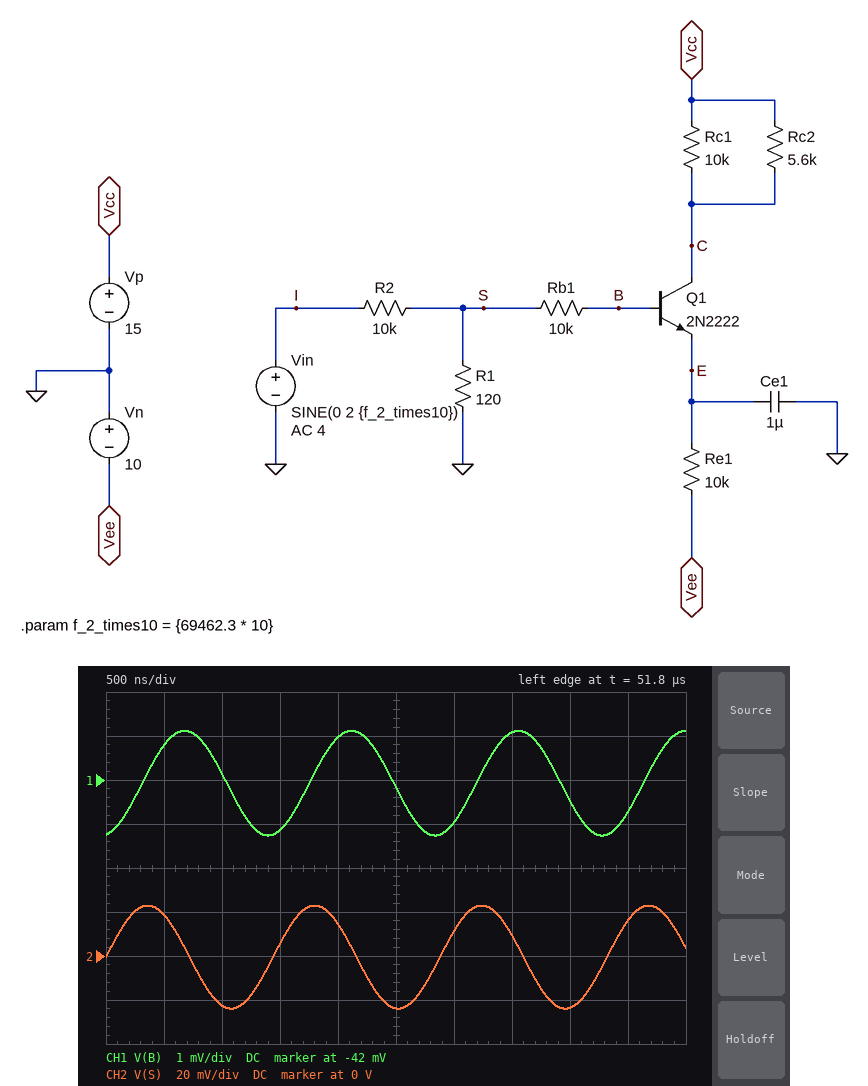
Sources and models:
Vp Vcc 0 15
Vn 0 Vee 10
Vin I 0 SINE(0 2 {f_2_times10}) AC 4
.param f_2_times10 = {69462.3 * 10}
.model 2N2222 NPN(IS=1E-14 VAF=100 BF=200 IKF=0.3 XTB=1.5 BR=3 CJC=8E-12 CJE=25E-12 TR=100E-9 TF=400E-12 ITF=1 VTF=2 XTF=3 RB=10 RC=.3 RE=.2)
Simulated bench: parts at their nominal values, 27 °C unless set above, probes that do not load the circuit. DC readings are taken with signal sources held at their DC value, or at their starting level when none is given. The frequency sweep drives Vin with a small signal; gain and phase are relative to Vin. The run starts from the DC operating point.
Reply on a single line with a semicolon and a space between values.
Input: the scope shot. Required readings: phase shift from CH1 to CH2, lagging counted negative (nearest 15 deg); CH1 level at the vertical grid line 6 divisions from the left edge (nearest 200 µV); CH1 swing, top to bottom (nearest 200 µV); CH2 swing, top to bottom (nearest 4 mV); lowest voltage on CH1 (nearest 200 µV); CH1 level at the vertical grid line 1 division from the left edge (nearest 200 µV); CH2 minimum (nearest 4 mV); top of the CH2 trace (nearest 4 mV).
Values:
75 deg; -43.0 mV; 2.4 mV; 48 mV; -43.2 mV; -41.2 mV; -24 mV; 24 mV
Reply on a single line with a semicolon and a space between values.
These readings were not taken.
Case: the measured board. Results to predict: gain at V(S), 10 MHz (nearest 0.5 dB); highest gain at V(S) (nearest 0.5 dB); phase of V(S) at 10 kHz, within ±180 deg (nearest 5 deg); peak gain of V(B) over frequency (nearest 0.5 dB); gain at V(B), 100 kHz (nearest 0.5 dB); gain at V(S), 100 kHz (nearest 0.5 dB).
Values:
-38.5 dB; -38.5 dB; 0 deg; -38.5 dB; -50.0 dB; -38.5 dB
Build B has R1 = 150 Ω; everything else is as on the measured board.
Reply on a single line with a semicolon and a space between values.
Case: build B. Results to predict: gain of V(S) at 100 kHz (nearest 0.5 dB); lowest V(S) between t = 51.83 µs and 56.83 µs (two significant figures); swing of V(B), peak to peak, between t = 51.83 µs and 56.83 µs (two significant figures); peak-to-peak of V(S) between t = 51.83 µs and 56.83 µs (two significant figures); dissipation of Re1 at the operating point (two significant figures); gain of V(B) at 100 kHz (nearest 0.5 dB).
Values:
-36.5 dB; -30 mV; 3.0 mV; 58 mV; 8.7 mW; -48.5 dB
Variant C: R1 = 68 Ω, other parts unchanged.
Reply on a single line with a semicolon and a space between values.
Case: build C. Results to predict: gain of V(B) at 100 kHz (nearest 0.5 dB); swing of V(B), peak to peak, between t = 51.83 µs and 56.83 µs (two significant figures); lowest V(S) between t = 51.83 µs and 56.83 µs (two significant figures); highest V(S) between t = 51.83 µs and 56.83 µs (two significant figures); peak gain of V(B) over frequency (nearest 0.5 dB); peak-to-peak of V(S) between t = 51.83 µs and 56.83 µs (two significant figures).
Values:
-55.0 dB; 1.4 mV; -14 mV; 13 mV; -43.5 dB; 27 mV
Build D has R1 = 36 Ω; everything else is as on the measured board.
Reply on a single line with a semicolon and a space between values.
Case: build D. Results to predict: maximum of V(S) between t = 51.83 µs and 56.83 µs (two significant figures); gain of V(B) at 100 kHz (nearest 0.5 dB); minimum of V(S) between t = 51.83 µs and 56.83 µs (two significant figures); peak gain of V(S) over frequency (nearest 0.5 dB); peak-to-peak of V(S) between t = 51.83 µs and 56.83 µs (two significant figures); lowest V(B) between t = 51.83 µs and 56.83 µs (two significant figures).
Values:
7.0 mV; -60.5 dB; -7.3 mV; -49.0 dB; 14 mV; -42 mV
